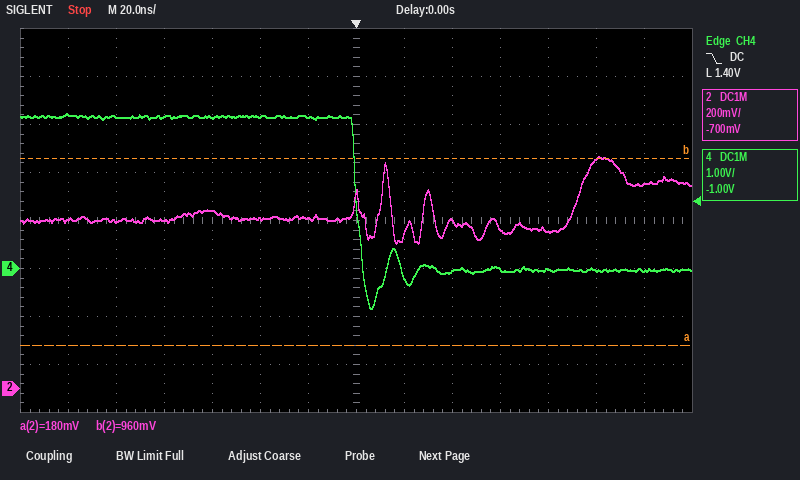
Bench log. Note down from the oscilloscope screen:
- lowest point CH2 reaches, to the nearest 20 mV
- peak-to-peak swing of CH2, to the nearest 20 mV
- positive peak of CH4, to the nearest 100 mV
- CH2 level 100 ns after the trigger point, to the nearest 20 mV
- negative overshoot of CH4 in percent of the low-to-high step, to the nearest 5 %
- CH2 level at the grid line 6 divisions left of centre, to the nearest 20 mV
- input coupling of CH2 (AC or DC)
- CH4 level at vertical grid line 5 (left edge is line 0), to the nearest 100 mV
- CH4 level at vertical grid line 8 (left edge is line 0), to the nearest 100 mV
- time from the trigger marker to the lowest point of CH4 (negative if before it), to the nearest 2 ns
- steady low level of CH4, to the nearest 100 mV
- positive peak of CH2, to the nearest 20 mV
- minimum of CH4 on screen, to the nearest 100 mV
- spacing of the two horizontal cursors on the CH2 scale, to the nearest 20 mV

600 mV
360 mV
3.2 V
960 mV
25 %
700 mV
DC
3.2 V
-200 mV
+6 ns
0.0 V
960 mV
-800 mV
780 mV
